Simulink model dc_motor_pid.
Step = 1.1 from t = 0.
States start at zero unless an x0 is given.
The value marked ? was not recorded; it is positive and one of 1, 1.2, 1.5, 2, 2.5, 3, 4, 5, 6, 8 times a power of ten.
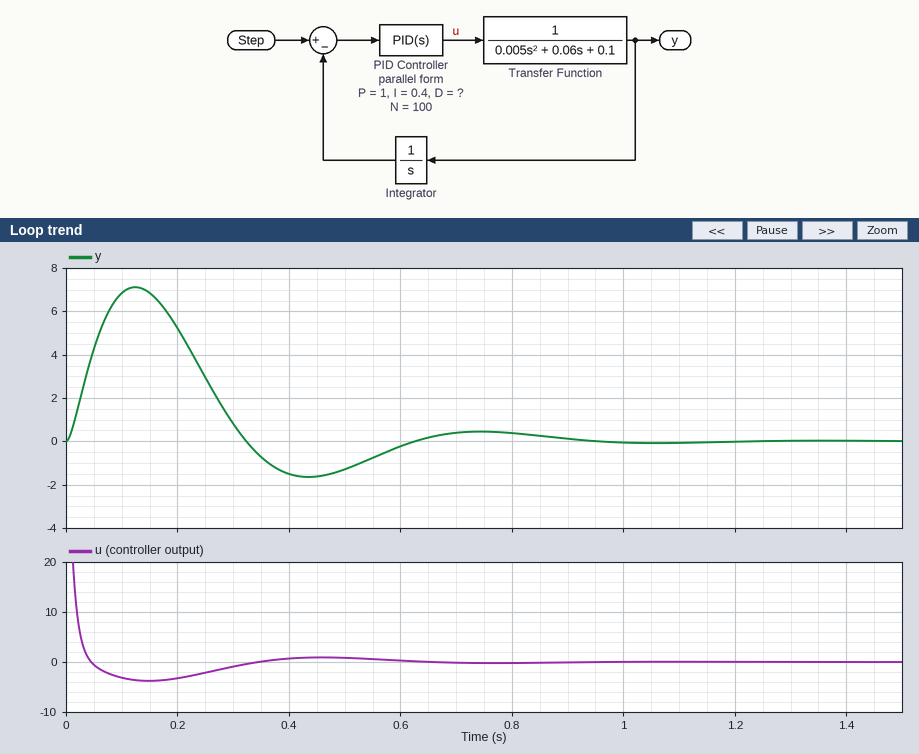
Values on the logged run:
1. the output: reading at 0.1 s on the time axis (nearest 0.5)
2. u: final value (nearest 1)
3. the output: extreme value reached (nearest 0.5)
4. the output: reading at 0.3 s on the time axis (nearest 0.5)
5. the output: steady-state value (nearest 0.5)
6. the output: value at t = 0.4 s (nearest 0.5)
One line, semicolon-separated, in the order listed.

7.0; 0; 7.0; 1.0; 0.0; -1.5
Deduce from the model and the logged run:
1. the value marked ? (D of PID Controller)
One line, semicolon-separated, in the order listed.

0.6
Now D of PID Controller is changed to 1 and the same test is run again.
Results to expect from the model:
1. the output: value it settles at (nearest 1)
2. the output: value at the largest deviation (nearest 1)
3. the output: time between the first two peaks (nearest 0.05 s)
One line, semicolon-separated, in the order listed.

0; 10; 0.45 s
